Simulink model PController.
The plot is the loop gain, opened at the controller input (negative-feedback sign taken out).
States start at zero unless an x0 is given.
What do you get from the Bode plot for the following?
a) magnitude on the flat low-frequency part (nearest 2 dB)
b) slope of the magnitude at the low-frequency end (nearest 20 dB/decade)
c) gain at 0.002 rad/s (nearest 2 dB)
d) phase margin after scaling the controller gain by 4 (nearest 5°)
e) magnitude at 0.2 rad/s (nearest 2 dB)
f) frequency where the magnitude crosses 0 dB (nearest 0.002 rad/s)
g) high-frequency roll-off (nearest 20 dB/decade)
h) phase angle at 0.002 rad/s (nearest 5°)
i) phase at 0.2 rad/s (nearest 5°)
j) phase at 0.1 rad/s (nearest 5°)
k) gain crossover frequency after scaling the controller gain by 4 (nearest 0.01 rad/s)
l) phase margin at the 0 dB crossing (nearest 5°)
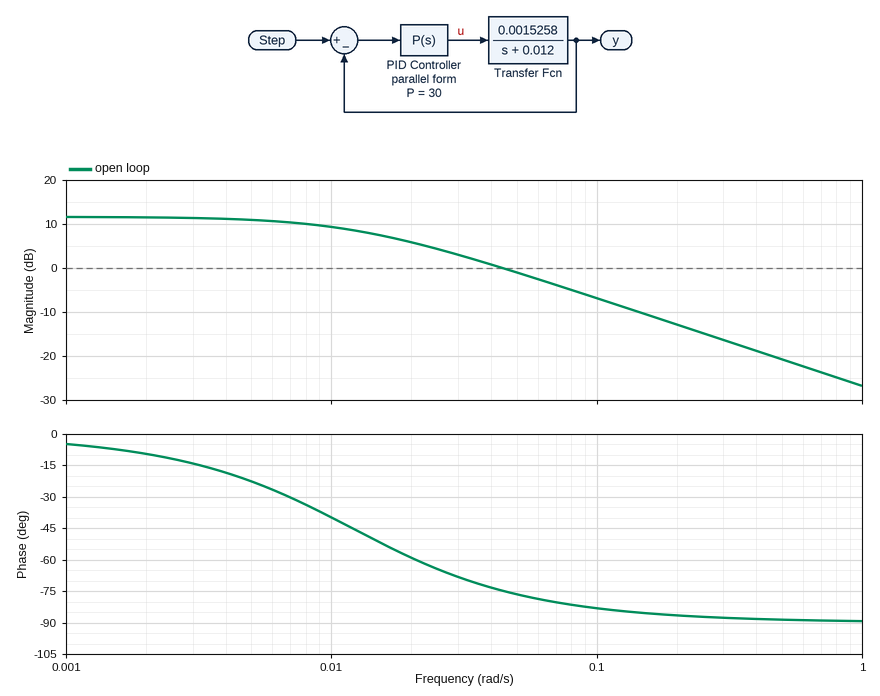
12 dB
0 dB/decade
12 dB
95°
-12 dB
0.044 rad/s
-20 dB/decade
-10°
-85°
-85°
0.18 rad/s
105°
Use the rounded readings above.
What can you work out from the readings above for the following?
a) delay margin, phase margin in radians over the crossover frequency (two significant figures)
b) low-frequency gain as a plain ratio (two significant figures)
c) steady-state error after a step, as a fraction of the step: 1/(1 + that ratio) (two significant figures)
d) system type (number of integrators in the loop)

42 s
4.0
0.20
0
